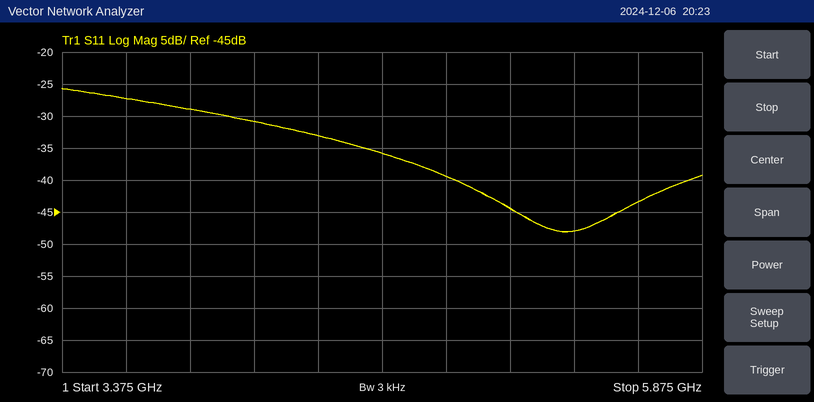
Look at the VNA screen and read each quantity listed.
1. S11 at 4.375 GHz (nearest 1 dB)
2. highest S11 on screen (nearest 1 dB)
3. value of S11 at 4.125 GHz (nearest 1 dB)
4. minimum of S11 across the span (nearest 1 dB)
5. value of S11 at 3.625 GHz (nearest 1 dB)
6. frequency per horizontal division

-33 dB
-26 dB
-31 dB
-48 dB
-27 dB
250 MHz
